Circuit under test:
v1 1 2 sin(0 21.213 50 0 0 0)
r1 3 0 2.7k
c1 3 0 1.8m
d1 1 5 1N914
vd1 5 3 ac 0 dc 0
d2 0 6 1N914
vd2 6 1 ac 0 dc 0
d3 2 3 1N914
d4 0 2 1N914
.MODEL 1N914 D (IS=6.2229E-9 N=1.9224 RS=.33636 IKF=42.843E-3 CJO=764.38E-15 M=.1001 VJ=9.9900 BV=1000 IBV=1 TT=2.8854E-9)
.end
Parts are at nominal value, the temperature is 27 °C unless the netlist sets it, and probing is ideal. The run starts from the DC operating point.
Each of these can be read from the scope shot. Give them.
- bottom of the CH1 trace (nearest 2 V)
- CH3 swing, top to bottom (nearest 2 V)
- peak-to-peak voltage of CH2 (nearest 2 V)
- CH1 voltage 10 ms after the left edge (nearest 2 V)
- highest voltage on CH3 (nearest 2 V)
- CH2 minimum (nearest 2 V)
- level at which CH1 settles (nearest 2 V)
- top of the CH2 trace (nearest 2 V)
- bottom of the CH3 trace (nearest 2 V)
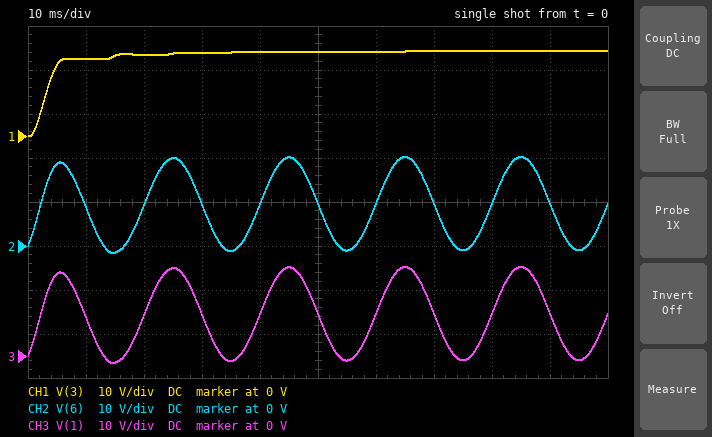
0 V
22 V
22 V
18 V
20 V
-2 V
20 V
20 V
-2 V
